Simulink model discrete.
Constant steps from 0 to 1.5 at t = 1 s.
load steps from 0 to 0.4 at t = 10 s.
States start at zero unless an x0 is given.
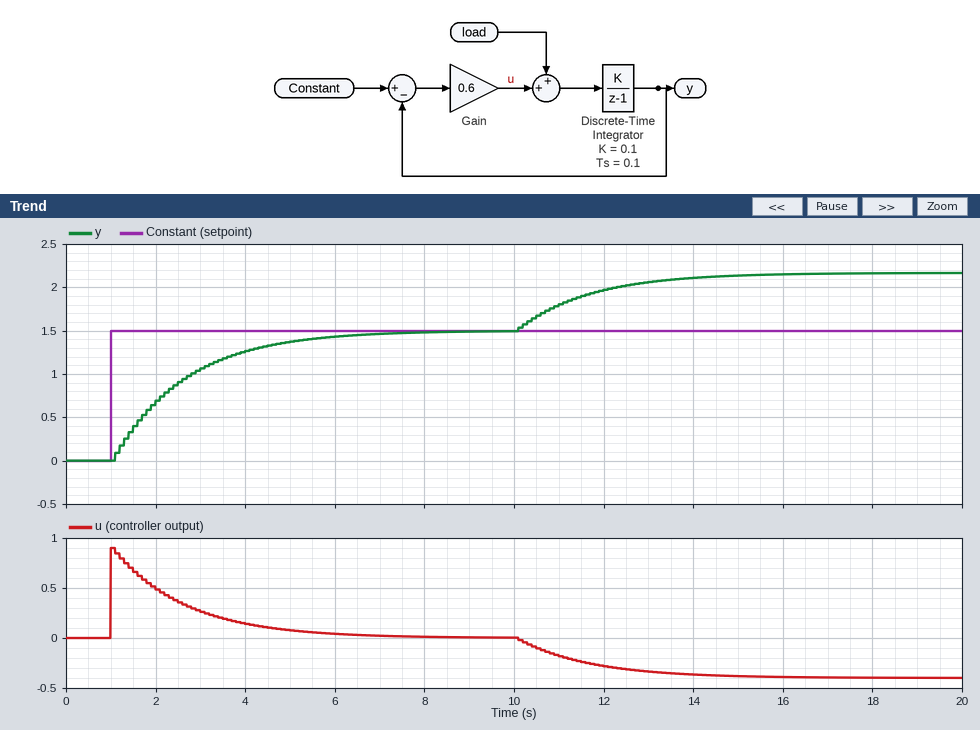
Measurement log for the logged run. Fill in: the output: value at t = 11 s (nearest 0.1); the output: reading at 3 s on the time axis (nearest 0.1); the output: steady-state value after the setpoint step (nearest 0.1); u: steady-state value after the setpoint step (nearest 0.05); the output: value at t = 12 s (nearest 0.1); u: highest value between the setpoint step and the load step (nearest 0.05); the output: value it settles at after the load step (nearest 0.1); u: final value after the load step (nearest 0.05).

1.8
1.1
1.5
0.00
2.0
0.90
2.2
-0.40
